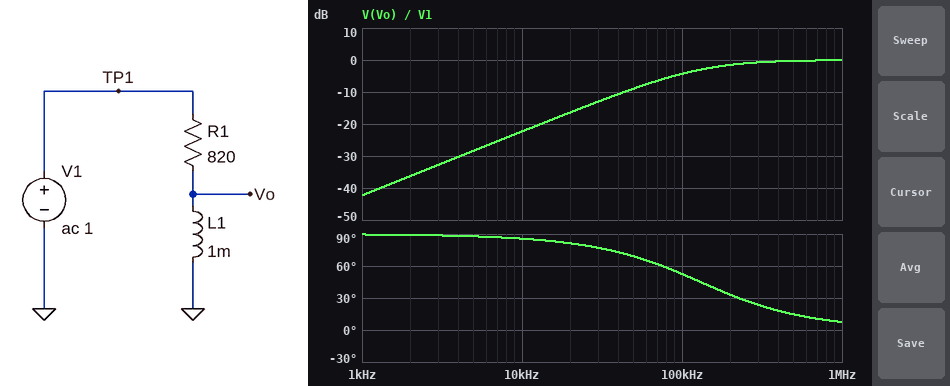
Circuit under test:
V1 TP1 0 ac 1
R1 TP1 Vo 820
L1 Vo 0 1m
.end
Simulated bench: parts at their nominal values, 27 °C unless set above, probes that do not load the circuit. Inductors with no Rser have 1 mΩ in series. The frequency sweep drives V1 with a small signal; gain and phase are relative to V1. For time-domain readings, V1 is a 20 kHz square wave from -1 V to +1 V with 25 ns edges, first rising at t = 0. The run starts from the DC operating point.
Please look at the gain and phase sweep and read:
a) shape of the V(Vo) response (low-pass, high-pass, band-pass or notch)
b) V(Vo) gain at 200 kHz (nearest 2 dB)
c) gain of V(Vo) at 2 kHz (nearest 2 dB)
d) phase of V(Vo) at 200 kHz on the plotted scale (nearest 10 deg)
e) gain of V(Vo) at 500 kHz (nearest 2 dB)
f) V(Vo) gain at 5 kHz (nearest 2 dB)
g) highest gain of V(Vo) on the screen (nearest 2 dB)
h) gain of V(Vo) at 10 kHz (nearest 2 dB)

high-pass
-2 dB
-36 dB
30 deg
0 dB
-28 dB
0 dB
-22 dB
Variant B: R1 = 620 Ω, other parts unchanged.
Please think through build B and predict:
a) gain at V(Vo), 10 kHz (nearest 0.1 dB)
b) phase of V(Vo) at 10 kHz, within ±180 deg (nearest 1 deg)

-19.9 dB
84 deg
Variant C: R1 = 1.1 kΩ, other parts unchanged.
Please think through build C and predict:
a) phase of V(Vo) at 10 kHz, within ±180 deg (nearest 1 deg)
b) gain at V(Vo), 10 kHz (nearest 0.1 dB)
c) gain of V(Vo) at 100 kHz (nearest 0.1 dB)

87 deg
-24.9 dB
-6.1 dB
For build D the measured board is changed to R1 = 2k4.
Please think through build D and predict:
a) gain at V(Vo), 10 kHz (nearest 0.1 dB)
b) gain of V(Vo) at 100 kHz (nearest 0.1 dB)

-31.6 dB
-11.9 dB
